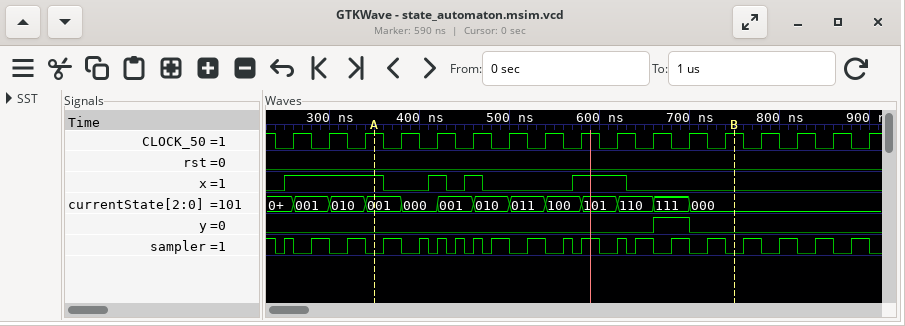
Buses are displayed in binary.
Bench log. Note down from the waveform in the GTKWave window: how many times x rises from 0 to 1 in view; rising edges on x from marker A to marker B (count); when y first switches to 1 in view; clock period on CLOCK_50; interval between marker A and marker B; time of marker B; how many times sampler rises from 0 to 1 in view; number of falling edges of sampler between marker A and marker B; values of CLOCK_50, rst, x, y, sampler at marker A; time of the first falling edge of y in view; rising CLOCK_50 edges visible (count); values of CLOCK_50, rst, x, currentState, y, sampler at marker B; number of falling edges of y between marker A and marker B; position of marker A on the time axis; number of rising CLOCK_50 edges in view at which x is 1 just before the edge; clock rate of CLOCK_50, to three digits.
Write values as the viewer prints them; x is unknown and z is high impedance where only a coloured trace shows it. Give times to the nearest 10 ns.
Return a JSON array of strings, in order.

["4", "3", "660 ns", "40 ns", "400 ns", "750 ns", "20", "13", "CLOCK_50=1, rst=0, x=1, y=0, sampler=0", "700 ns", "17", "CLOCK_50=1, rst=0, x=0, currentState=000, y=0, sampler=0", "1", "350 ns", "7", "25.0 MHz"]
